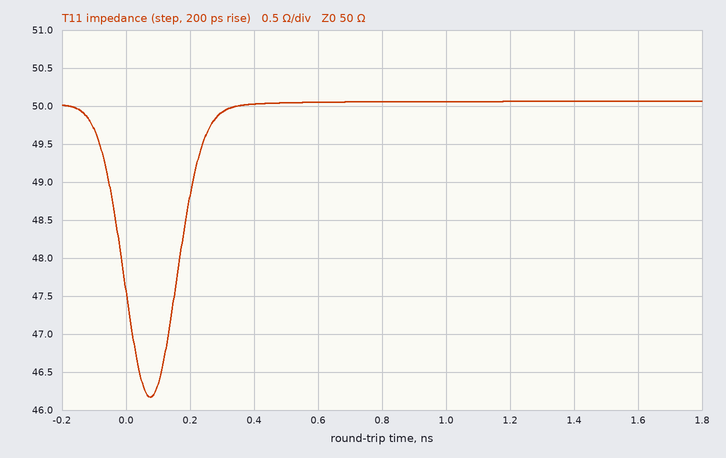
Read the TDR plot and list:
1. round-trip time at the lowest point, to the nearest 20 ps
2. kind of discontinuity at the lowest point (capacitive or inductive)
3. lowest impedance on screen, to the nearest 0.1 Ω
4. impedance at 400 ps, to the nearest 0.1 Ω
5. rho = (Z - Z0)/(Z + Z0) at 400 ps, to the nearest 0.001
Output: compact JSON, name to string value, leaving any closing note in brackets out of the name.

{"round-trip time at the lowest point, to the nearest 20 ps": "80 ps", "kind of discontinuity at the lowest point": "capacitive", "lowest impedance on screen, to the nearest 0.1 Ω": "46.2 Ω", "impedance at 400 ps, to the nearest 0.1 Ω": "50.0 Ω", "rho = (Z - Z0)/(Z + Z0) at 400 ps, to the nearest 0.001": "0.000"}
